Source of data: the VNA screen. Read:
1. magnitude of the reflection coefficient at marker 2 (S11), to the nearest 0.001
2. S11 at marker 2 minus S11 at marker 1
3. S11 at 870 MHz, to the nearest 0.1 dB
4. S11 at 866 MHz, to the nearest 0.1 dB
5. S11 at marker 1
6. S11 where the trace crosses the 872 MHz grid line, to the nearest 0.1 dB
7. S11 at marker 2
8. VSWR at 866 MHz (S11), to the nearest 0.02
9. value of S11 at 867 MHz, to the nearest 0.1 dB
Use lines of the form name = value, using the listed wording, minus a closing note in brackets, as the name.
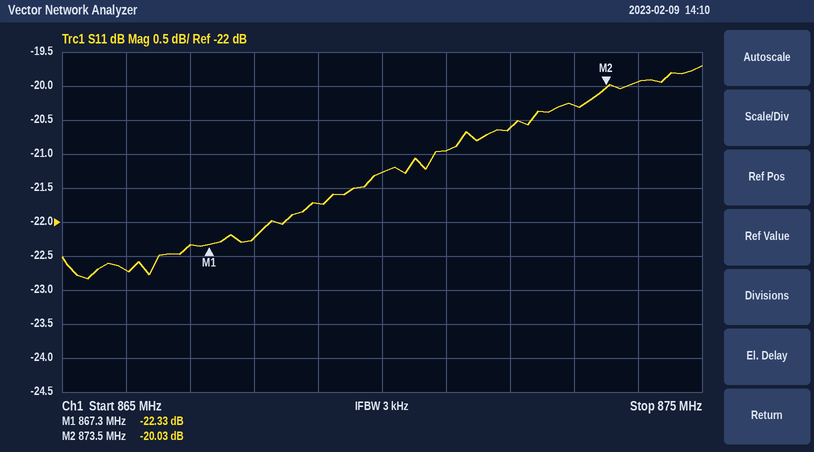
magnitude of the reflection coefficient at marker 2 (S11), to the nearest 0.001 = 0.100
S11 at marker 2 minus S11 at marker 1 = 2.30 dB
S11 at 870 MHz, to the nearest 0.1 dB = -21.3 dB
S11 at 866 MHz, to the nearest 0.1 dB = -22.7 dB
S11 at marker 1 = -22.33 dB
S11 where the trace crosses the 872 MHz grid line, to the nearest 0.1 dB = -20.6 dB
S11 at marker 2 = -20.03 dB
VSWR at 866 MHz (S11), to the nearest 0.02 = 1.16
value of S11 at 867 MHz, to the nearest 0.1 dB = -22.3 dB
